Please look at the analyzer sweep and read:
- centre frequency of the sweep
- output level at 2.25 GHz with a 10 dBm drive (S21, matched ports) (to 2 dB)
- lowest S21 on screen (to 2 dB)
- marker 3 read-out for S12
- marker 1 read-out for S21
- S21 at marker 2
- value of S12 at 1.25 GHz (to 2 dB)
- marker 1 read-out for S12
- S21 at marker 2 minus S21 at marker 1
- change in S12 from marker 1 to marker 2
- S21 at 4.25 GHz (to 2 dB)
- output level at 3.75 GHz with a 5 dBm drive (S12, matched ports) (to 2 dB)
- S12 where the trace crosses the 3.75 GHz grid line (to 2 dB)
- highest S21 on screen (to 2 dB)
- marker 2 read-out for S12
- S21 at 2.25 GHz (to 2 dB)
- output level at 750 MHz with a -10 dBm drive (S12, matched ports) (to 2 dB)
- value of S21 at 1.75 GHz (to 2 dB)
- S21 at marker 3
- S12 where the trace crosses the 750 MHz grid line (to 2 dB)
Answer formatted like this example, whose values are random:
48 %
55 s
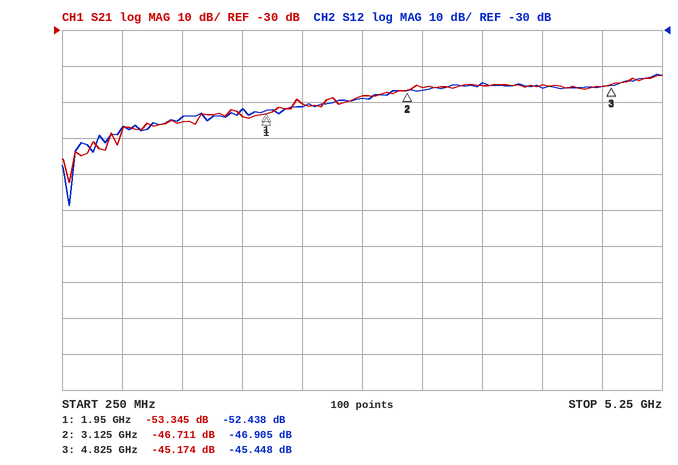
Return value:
2.75 GHz
-40 dBm
-72 dB
-45.448 dB
-53.345 dB
-46.711 dB
-54 dB
-52.438 dB
6.634 dB
5.533 dB
-46 dB
-40 dBm
-44 dB
-42 dB
-46.905 dB
-50 dB
-68 dBm
-54 dB
-45.174 dB
-58 dB
